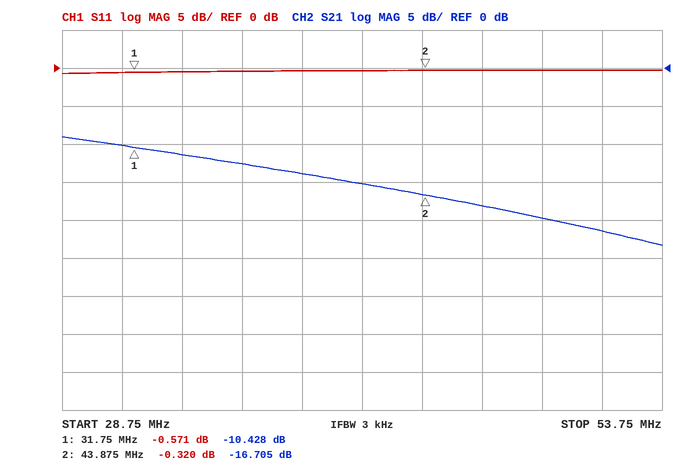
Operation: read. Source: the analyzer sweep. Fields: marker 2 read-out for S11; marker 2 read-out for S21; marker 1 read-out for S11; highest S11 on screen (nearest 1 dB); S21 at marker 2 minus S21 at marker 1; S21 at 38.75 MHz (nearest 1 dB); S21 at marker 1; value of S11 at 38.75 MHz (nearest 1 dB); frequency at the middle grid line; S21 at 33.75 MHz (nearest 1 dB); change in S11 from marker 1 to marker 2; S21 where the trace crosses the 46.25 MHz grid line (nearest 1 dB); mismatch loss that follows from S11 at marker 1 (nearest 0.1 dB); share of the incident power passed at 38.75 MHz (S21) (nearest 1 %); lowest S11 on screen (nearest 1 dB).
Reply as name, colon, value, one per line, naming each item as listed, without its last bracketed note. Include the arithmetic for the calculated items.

marker 2 read-out for S11: -0.320 dB
marker 2 read-out for S21: -16.705 dB
marker 1 read-out for S11: -0.571 dB
highest S11 on screen: 0 dB
S21 at marker 2 minus S21 at marker 1: -16.705 − (-10.428) = -6.277 dB
S21 at 38.75 MHz: -14 dB
S21 at marker 1: -10.428 dB
value of S11 at 38.75 MHz: 0 dB
frequency at the middle grid line: 41.25 MHz
S21 at 33.75 MHz: -11 dB
change in S11 from marker 1 to marker 2: -0.32 − (-0.571) = 0.251 dB
S21 where the trace crosses the 46.25 MHz grid line: -18 dB
mismatch loss that follows from S11 at marker 1: −10 log10(1 − 10^(-0.571/10)) ≈ 9.1 dB
share of the incident power passed at 38.75 MHz (S21): 10^(-14/10) ≈ 4 %
lowest S11 on screen: -1 dB
